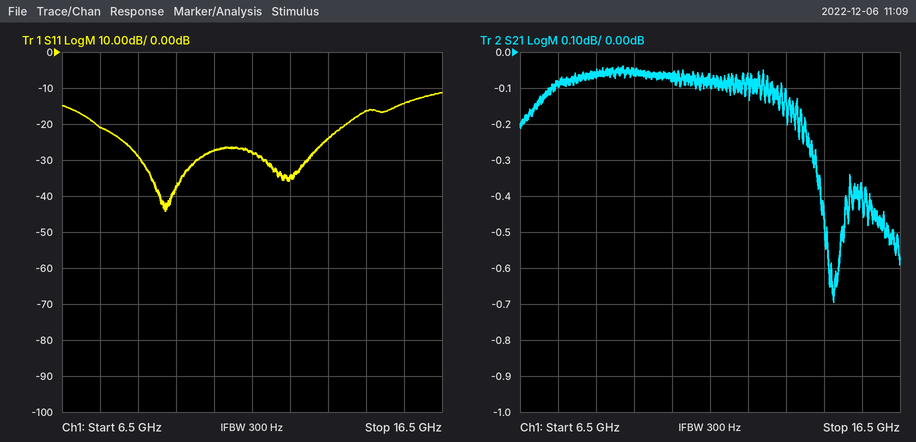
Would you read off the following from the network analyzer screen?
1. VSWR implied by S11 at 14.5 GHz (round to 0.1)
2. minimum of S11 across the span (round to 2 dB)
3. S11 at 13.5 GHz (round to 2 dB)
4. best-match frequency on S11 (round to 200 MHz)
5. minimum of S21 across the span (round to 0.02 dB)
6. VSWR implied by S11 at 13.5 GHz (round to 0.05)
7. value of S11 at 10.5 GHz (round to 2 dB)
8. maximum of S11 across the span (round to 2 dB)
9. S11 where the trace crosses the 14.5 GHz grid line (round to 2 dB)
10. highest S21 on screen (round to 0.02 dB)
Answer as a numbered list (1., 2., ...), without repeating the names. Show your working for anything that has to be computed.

1. |Γ| = 10^(-16/20) = 0.1585; VSWR = (1 + 0.1585)/(1 − 0.1585) ≈ 1.4
2. -44 dB
3. -24 dB
4. 9.2 GHz
5. -0.70 dB
6. |Γ| = 10^(-24/20) = 0.0631; VSWR = (1 + 0.0631)/(1 − 0.0631) ≈ 1.13, so 1.15 to the nearest 0.05
7. -28 dB
8. -12 dB
9. -16 dB
10. -0.04 dB
